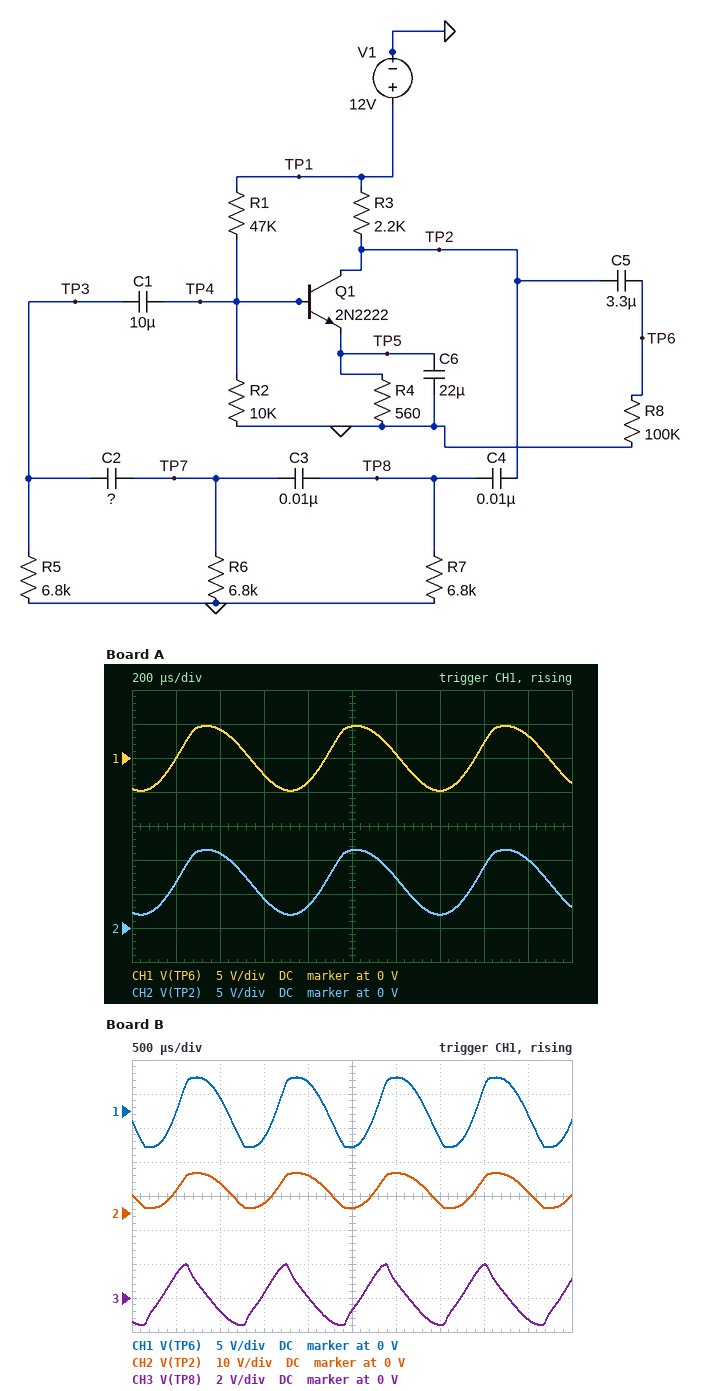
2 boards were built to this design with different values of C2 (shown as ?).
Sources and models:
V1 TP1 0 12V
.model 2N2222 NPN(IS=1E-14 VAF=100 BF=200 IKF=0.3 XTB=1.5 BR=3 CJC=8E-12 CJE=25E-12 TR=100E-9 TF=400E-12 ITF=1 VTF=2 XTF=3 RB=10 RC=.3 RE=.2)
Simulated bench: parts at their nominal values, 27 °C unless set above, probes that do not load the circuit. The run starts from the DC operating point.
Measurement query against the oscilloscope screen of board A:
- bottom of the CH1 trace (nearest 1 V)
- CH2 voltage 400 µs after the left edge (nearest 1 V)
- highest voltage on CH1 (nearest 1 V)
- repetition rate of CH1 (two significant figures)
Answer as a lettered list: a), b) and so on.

a) -5 V
b) 11 V
c) 5 V
d) 1.5 kHz
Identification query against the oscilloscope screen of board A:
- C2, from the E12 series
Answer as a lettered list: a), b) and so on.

a) 3.3 nF
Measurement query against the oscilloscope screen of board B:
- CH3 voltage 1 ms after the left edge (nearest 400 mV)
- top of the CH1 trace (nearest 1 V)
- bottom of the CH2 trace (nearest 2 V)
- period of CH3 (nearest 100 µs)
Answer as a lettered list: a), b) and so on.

a) -800 mV
b) 5 V
c) 2 V
d) 1.1 ms
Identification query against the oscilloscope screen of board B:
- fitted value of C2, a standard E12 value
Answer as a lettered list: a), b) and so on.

a) 18 nF
